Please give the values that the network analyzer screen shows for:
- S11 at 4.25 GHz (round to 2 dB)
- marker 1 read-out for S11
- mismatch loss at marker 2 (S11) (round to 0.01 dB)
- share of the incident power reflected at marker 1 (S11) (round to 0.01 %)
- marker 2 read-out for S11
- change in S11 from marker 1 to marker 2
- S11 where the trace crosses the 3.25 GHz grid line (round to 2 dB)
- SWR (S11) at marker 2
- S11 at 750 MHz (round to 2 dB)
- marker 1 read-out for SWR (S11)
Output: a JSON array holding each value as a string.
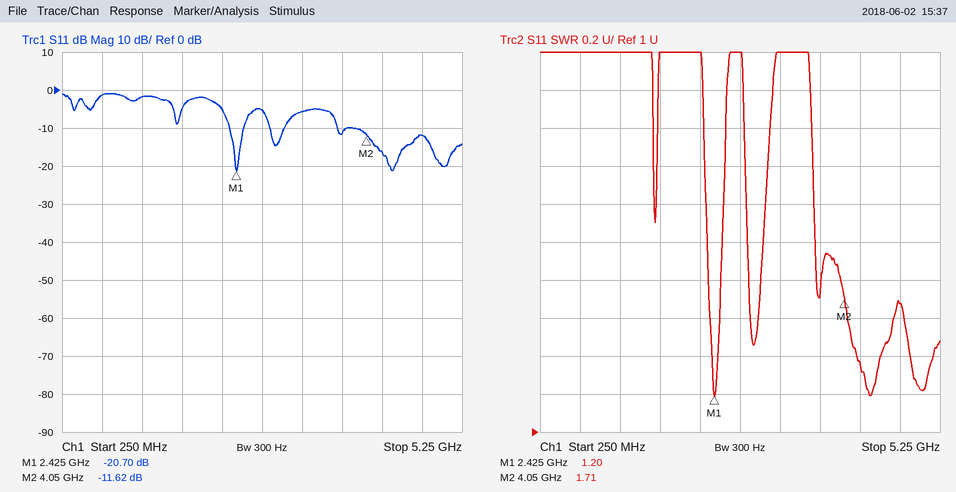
["-16 dB", "-20.70 dB", "0.31 dB", "0.85 %", "-11.62 dB", "9.08 dB", "-6 dB", "1.71", "-2 dB", "1.20"]
